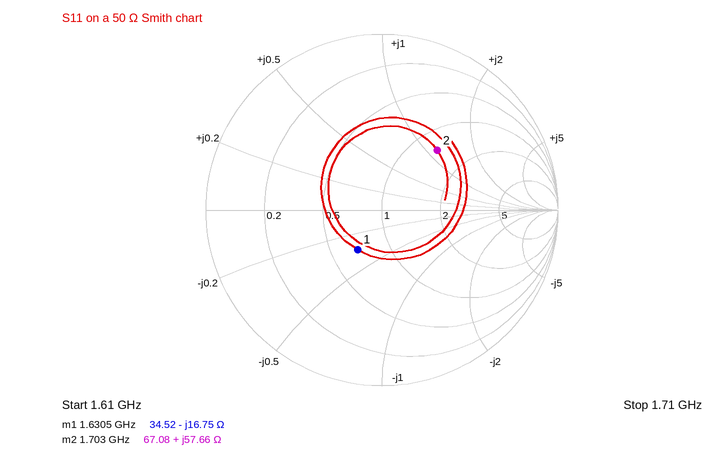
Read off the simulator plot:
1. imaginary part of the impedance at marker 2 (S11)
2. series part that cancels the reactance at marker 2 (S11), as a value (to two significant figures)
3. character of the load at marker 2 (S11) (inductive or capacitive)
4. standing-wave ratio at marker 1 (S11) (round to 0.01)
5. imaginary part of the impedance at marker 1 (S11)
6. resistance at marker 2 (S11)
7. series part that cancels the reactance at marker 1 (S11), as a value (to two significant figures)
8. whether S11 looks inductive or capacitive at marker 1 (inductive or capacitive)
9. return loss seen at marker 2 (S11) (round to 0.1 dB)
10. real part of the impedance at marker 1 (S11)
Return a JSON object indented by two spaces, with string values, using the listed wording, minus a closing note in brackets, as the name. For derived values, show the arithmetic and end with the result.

{
  "imaginary part of the impedance at marker 2": "+57.66 Ω",
  "series part that cancels the reactance at marker 2 (S11), as a value": "C = 1/(2π × 1.703 GHz × 57.66 Ω) ≈ 1.6 pF",
  "character of the load at marker 2 (S11)": "inductive",
  "standing-wave ratio at marker 1 (S11)": "1.72",
  "imaginary part of the impedance at marker 1": "-16.75 Ω",
  "resistance at marker 2": "67.08 Ω",
  "series part that cancels the reactance at marker 1 (S11), as a value": "L = 16.75 Ω/(2π × 1.6305 GHz) ≈ 1.6 nH",
  "whether S11 looks inductive or capacitive at marker 1": "capacitive",
  "return loss seen at marker 2 (S11)": "6.7 dB",
  "real part of the impedance at marker 1": "34.52 Ω"
}
